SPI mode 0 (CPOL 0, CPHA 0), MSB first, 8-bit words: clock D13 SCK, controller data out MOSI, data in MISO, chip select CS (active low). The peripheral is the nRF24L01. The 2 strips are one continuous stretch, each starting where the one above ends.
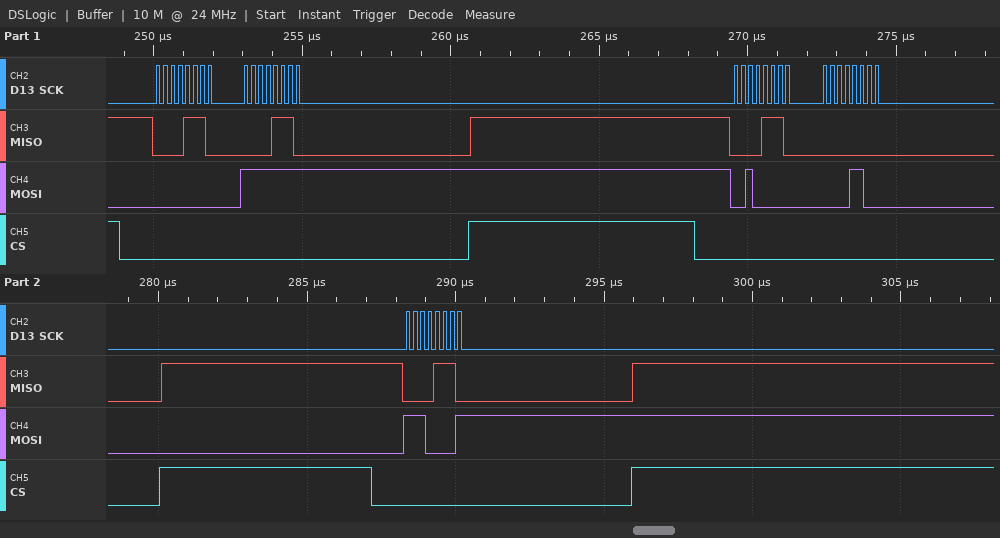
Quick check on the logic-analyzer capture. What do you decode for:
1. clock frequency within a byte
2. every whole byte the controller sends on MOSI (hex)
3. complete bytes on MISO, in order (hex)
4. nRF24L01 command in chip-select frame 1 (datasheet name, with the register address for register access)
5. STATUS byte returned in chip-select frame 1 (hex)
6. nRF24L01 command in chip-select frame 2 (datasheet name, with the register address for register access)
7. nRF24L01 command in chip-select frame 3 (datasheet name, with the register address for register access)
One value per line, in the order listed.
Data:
4 MHz
00 FF 20 0C E1
0E 0E 0E 00 0E
R_REGISTER 0x00
0x0E
W_REGISTER 0x00
FLUSH_TX
